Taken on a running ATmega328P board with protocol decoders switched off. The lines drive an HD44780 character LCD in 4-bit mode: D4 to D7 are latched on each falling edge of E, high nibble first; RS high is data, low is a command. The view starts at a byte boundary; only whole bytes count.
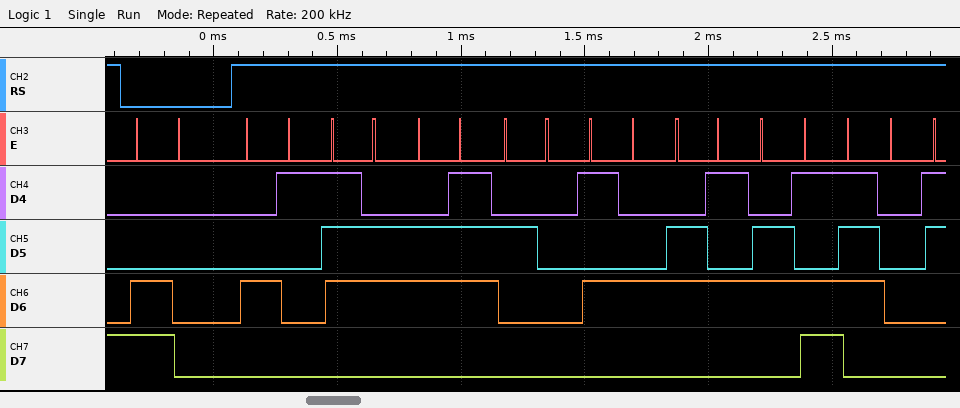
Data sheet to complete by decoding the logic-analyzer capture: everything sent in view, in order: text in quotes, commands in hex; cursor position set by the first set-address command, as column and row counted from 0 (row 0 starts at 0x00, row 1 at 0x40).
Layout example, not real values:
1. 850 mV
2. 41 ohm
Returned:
1. 0xC0 "Avg Temp"
2. column 0, row 1
